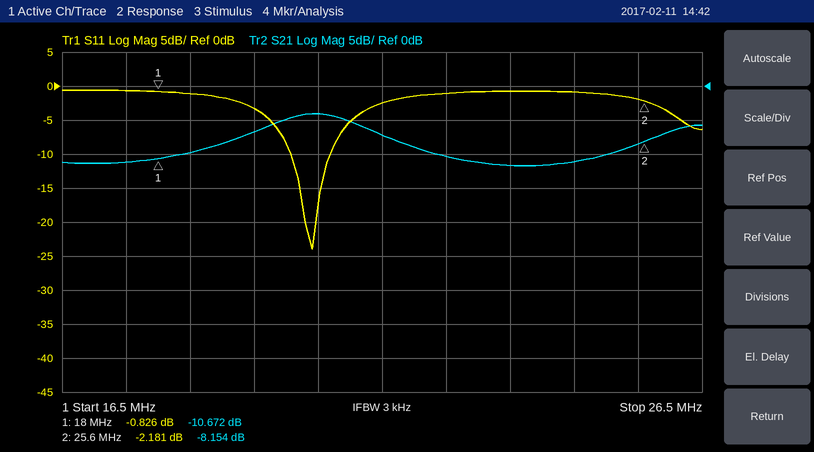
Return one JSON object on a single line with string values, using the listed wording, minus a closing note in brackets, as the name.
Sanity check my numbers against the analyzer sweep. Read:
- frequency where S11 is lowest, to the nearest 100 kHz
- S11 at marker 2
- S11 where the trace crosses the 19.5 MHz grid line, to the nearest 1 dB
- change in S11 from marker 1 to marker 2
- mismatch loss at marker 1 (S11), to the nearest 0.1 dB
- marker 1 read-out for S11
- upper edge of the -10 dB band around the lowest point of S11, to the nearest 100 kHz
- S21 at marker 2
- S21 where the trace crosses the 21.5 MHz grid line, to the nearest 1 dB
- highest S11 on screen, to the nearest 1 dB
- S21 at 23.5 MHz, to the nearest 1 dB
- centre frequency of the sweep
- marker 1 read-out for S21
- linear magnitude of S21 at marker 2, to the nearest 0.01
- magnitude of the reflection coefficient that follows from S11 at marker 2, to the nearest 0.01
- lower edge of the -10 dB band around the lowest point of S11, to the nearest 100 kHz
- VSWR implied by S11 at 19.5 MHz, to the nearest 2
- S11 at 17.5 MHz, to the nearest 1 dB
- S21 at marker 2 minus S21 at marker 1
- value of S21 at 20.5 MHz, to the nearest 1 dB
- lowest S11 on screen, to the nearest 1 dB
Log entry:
{"frequency where S11 is lowest, to the nearest 100 kHz": "20.4 MHz", "S11 at marker 2": "-2.181 dB", "S11 where the trace crosses the 19.5 MHz grid line, to the nearest 1 dB": "-3 dB", "change in S11 from marker 1 to marker 2": "-1.355 dB", "mismatch loss at marker 1 (S11), to the nearest 0.1 dB": "7.6 dB", "marker 1 read-out for S11": "-0.826 dB", "upper edge of the -10 dB band around the lowest point of S11, to the nearest 100 kHz": "20.7 MHz", "S21 at marker 2": "-8.154 dB", "S21 where the trace crosses the 21.5 MHz grid line, to the nearest 1 dB": "-7 dB", "highest S11 on screen, to the nearest 1 dB": "-1 dB", "S21 at 23.5 MHz, to the nearest 1 dB": "-12 dB", "centre frequency of the sweep": "21.5 MHz", "marker 1 read-out for S21": "-10.672 dB", "linear magnitude of S21 at marker 2, to the nearest 0.01": "0.39", "magnitude of the reflection coefficient that follows from S11 at marker 2, to the nearest 0.01": "0.78", "lower edge of the -10 dB band around the lowest point of S11, to the nearest 100 kHz": "20.1 MHz", "VSWR implied by S11 at 19.5 MHz, to the nearest 2": "6", "S11 at 17.5 MHz, to the nearest 1 dB": "-1 dB", "S21 at marker 2 minus S21 at marker 1": "2.518 dB", "value of S21 at 20.5 MHz, to the nearest 1 dB": "-4 dB", "lowest S11 on screen, to the nearest 1 dB": "-24 dB"}
